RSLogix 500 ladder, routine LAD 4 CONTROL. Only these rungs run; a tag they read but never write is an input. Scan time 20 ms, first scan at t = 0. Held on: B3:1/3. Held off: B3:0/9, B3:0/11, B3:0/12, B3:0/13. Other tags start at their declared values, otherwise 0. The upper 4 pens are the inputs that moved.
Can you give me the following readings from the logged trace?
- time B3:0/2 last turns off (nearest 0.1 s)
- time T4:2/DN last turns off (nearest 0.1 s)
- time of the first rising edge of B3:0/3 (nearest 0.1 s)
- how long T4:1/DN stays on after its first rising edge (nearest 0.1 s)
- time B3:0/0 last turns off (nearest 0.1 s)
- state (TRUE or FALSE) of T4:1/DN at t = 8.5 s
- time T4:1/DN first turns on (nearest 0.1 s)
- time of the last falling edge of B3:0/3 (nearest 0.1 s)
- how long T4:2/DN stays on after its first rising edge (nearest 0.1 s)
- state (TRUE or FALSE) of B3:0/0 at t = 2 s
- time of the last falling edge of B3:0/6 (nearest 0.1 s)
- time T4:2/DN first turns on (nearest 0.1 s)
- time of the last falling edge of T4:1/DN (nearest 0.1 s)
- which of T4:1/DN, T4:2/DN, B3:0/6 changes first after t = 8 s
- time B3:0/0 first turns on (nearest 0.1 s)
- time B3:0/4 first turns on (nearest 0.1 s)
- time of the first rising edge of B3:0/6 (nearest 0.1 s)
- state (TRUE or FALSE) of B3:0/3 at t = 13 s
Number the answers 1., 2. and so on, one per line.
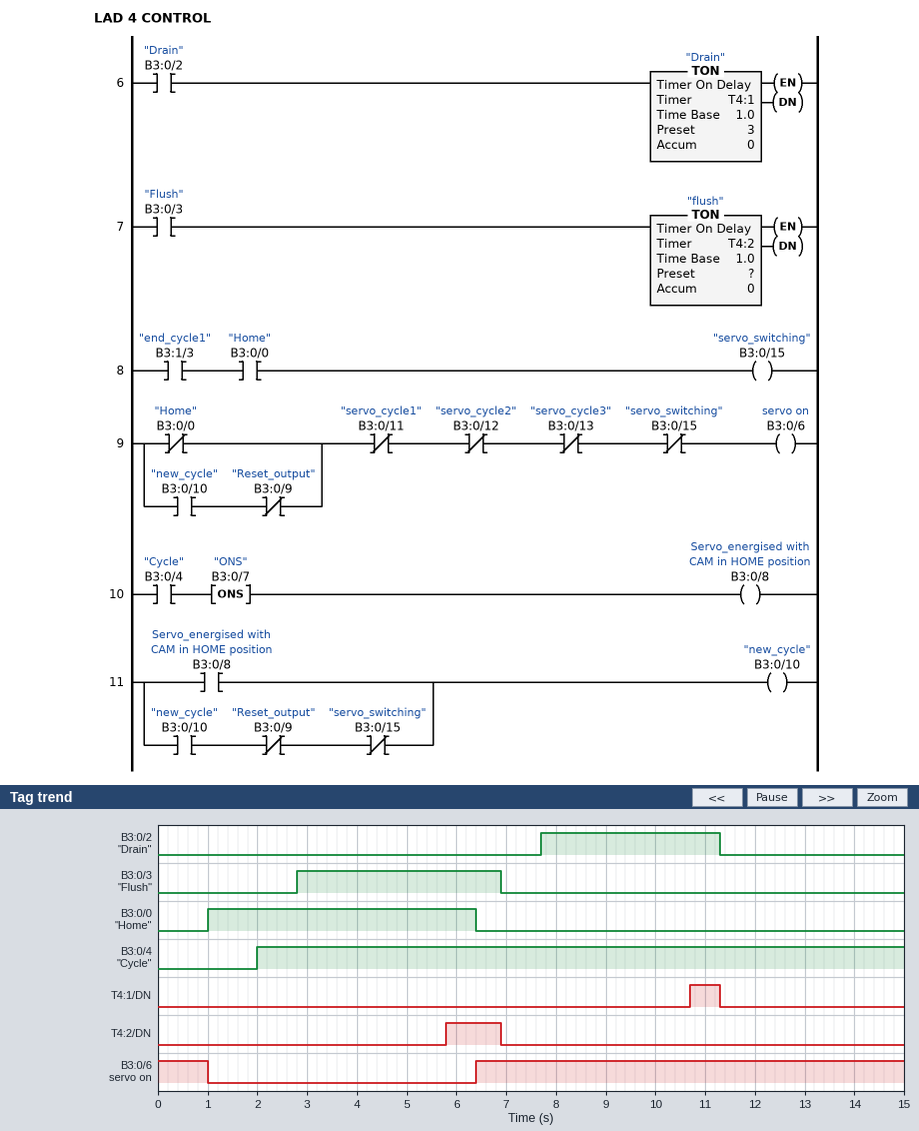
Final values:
1. 11.3 s
2. 6.9 s
3. 2.8 s
4. 0.6 s
5. 6.4 s
6. FALSE
7. 10.7 s
8. 6.9 s
9. 1.1 s
10. TRUE
11. 1.0 s
12. 5.8 s
13. 11.3 s
14. T4:1/DN
15. 1.0 s
16. 2.0 s
17. 6.4 s
18. FALSE
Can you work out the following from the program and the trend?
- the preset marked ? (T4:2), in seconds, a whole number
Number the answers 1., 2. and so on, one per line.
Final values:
1. 3 s
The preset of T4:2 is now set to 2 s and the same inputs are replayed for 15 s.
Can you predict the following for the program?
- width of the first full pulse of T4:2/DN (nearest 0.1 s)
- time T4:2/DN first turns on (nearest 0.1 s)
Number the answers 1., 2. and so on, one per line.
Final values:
1. 2.1 s
2. 4.8 s
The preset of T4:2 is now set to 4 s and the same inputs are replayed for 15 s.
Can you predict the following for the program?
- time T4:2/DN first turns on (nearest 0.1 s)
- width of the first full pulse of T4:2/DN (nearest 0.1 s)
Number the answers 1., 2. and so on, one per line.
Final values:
1. 6.8 s
2. 0.1 s
